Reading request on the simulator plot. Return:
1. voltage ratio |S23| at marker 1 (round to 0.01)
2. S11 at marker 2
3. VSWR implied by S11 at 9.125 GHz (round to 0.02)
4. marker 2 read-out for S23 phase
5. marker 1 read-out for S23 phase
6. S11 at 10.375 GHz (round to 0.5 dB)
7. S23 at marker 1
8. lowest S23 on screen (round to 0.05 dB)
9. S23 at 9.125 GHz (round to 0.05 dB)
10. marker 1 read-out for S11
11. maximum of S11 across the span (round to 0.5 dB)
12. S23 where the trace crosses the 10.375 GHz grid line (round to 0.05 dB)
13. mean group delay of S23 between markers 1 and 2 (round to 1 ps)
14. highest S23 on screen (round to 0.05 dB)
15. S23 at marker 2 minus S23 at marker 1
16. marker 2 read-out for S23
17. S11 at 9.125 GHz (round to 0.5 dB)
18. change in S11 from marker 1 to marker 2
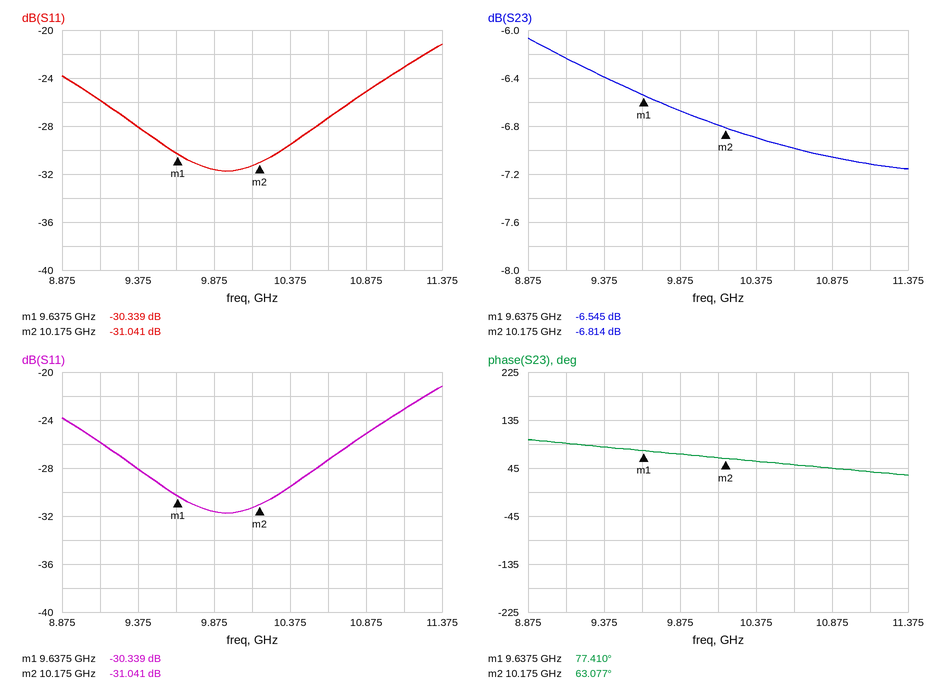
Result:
0.47
-31.041 dB
1.10
63.077°
77.410°
-29.5 dB
-6.545 dB
-7.15 dB
-6.25 dB
-30.339 dB
-21.0 dB
-6.90 dB
74 ps
-6.05 dB
-0.269 dB
-6.814 dB
-26.0 dB
-0.702 dB
